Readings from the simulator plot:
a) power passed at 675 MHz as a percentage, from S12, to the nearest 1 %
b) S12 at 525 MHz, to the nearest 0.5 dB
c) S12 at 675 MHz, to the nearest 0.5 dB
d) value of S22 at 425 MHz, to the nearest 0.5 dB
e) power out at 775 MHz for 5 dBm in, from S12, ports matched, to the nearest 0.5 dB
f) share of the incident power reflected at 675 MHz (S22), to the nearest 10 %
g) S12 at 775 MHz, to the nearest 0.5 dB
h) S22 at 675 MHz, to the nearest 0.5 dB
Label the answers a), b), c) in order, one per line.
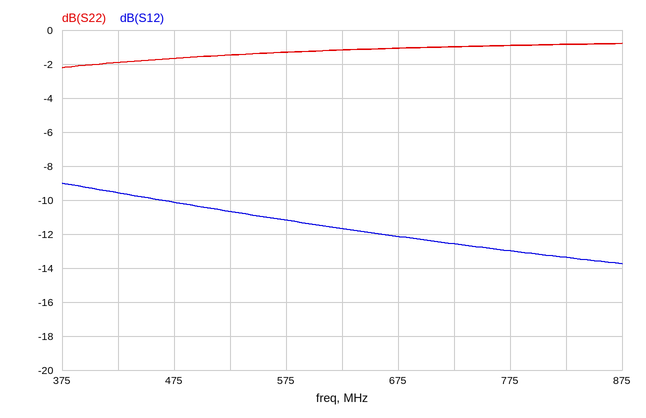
a) 6 %
b) -10.5 dB
c) -12.0 dB
d) -2.0 dB
e) -8.0 dBm
f) 80 %
g) -13.0 dB
h) -1.0 dB
